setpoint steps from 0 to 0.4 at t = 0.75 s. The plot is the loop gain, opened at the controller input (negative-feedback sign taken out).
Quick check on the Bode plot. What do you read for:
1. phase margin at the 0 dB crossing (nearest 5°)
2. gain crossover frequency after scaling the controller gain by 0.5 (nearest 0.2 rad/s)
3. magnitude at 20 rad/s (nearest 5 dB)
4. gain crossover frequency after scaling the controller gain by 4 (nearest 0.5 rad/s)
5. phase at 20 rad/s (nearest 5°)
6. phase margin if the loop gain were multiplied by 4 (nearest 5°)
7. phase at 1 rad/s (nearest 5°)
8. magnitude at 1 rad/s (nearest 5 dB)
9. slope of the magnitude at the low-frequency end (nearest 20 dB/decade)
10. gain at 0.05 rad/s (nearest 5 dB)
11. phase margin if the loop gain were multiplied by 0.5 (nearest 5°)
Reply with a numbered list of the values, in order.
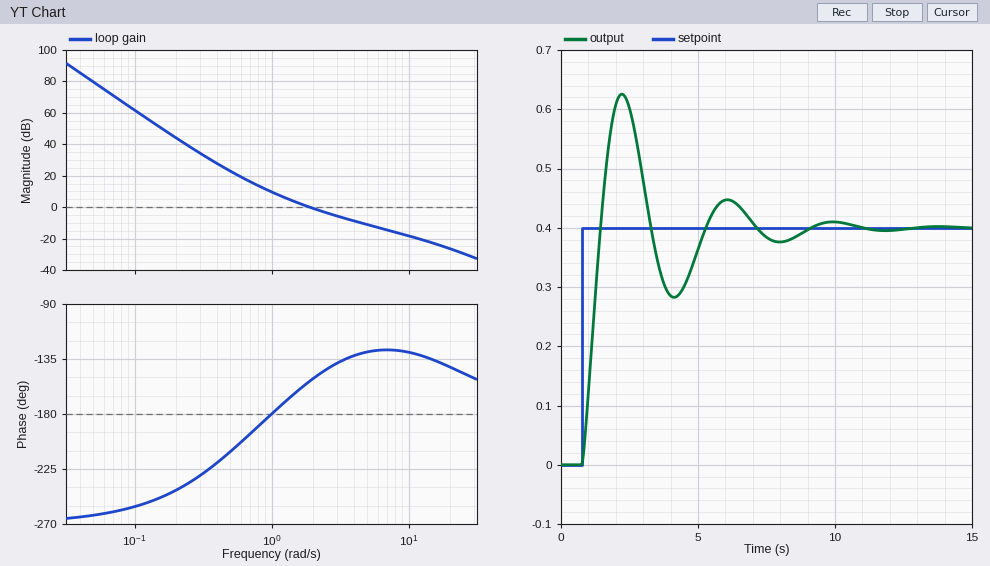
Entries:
1. 25°
2. 1.2 rad/s
3. -25 dB
4. 5.5 rad/s
5. -140°
6. 50°
7. -180°
8. 10 dB
9. -60 dB/decade
10. 80 dB
11. 10°
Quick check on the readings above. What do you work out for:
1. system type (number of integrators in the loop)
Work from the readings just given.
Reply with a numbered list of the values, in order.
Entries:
1. 3
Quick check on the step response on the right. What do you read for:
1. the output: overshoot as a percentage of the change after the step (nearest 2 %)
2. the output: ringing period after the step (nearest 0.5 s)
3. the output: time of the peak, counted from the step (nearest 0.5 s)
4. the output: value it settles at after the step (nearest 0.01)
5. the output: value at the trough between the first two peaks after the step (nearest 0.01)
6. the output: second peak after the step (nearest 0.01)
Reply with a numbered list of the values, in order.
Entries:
1. 56 %
2. 4.0 s
3. 1.5 s
4. 0.40
5. 0.28
6. 0.45
